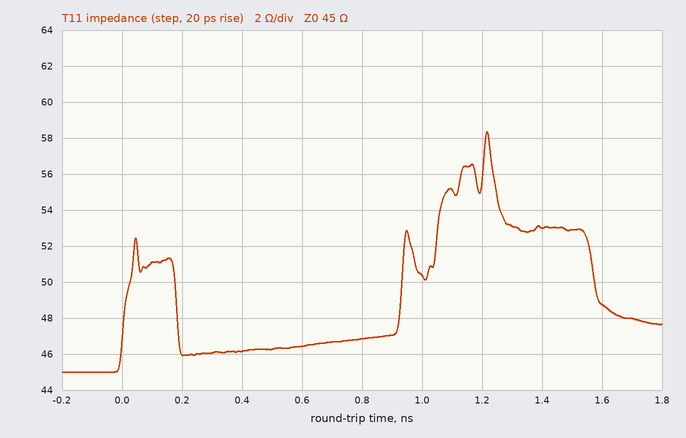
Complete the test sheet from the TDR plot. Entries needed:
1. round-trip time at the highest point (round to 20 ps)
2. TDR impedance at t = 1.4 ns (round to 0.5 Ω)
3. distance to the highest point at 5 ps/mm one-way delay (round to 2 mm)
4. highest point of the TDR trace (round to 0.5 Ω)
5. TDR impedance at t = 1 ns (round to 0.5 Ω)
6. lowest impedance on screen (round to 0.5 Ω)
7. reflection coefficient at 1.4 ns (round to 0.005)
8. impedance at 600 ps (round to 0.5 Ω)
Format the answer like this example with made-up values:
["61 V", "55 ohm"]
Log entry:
["1.22 ns", "53.0 Ω", "122 mm", "58.5 Ω", "50.5 Ω", "45.0 Ω", "+0.080", "46.5 Ω"]
